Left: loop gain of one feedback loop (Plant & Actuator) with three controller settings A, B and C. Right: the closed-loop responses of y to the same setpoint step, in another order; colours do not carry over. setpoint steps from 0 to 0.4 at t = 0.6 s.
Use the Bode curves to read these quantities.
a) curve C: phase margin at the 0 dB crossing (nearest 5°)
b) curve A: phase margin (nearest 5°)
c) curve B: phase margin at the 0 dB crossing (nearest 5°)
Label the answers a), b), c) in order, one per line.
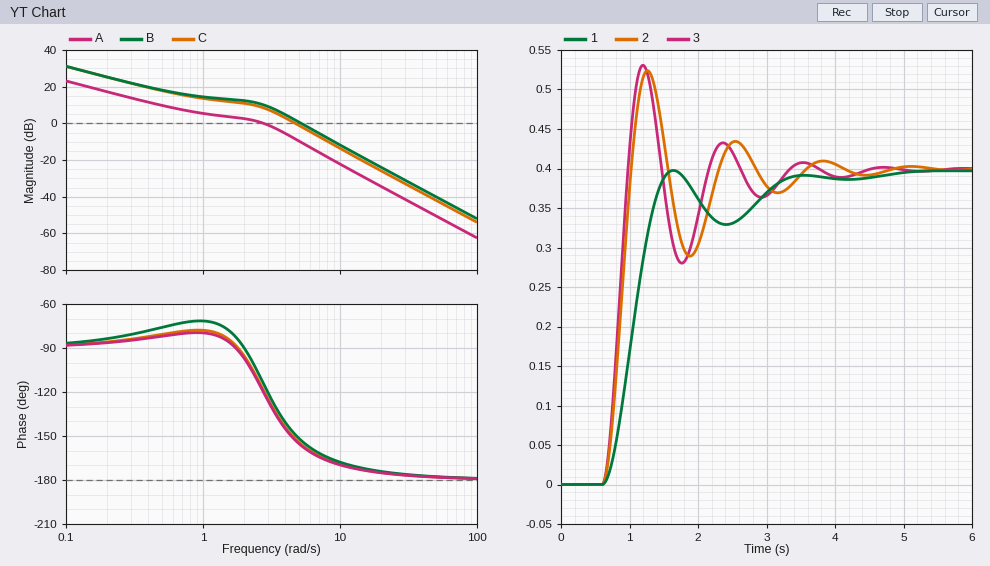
a) 30°
b) 60°
c) 25°
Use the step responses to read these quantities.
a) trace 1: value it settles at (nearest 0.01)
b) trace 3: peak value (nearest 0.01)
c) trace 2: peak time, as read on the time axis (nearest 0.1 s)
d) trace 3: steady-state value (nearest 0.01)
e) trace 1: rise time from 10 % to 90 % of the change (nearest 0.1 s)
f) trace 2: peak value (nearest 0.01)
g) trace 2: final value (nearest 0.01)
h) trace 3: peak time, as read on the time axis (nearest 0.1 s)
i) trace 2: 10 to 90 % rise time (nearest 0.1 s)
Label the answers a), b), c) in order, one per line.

a) 0.40
b) 0.53
c) 1.3 s
d) 0.40
e) 0.6 s
f) 0.52
g) 0.40
h) 1.2 s
i) 0.3 s
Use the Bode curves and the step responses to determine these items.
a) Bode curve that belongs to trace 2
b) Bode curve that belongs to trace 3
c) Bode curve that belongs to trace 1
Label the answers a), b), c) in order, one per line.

a) C
b) B
c) A
